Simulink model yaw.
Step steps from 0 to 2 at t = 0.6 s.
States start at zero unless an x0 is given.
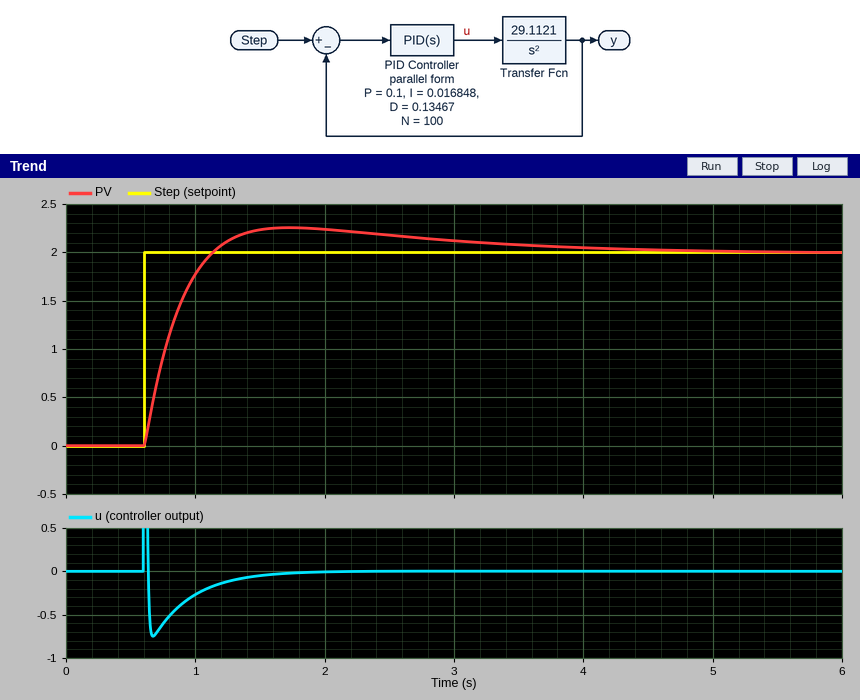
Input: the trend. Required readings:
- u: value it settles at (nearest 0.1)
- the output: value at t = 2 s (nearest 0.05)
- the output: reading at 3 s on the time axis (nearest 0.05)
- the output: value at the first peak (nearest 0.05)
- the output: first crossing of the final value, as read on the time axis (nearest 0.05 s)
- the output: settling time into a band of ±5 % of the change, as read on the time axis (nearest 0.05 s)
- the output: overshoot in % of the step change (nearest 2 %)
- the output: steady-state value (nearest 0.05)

0.0
2.25
2.10
2.25
1.15 s
3.20 s
12 %
2.00
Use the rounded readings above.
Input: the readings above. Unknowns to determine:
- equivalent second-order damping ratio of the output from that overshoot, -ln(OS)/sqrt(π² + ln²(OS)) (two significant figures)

0.56
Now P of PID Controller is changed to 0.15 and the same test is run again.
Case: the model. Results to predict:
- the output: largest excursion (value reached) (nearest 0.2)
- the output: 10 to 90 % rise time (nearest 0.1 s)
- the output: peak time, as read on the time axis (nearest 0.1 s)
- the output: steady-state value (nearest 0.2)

2.4
0.3 s
1.6 s
2.0
